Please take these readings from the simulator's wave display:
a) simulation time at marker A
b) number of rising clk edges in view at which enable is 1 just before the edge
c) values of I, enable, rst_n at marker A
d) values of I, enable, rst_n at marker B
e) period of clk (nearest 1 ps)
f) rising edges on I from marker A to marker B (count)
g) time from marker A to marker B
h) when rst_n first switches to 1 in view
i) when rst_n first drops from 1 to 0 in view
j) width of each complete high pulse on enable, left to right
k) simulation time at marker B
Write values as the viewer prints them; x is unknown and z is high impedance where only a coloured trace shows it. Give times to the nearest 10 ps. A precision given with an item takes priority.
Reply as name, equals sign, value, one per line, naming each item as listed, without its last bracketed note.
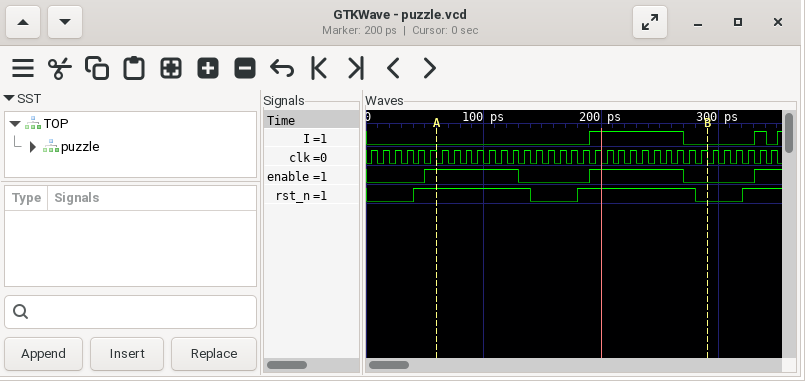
simulation time at marker A = 60 ps
number of rising clk edges in view at which enable is 1 just before the edge = 18
values of I, enable, rst_n at marker A = I=0, enable=1, rst_n=1
values of I, enable, rst_n at marker B = I=0, enable=0, rst_n=0
period of clk = 10 ps
rising edges on I from marker A to marker B = 1
time from marker A to marker B = 230 ps
when rst_n first switches to 1 in view = 40 ps
when rst_n first drops from 1 to 0 in view = 140 ps
width of each complete high pulse on enable, left to right = 80 ps, 80 ps
simulation time at marker B = 290 ps
